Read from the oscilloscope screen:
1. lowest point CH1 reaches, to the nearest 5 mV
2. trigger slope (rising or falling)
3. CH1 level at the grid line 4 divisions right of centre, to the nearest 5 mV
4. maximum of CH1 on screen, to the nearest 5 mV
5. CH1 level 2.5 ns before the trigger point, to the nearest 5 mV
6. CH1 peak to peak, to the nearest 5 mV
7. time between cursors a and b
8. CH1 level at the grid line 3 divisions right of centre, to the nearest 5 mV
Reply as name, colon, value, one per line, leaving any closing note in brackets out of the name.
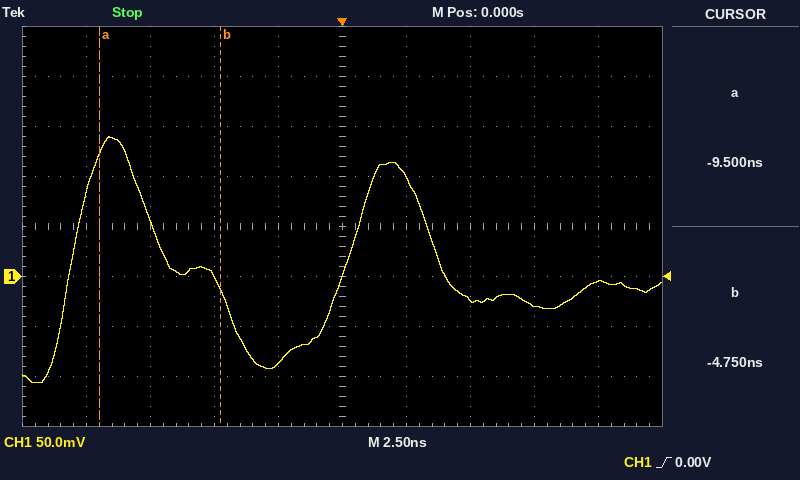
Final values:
lowest point CH1 reaches, to the nearest 5 mV: -105 mV
trigger slope: rising
CH1 level at the grid line 4 divisions right of centre, to the nearest 5 mV: -5 mV
maximum of CH1 on screen, to the nearest 5 mV: 140 mV
CH1 level 2.5 ns before the trigger point, to the nearest 5 mV: -85 mV
CH1 peak to peak, to the nearest 5 mV: 245 mV
time between cursors a and b: 4.75 ns
CH1 level at the grid line 3 divisions right of centre, to the nearest 5 mV: -30 mV
